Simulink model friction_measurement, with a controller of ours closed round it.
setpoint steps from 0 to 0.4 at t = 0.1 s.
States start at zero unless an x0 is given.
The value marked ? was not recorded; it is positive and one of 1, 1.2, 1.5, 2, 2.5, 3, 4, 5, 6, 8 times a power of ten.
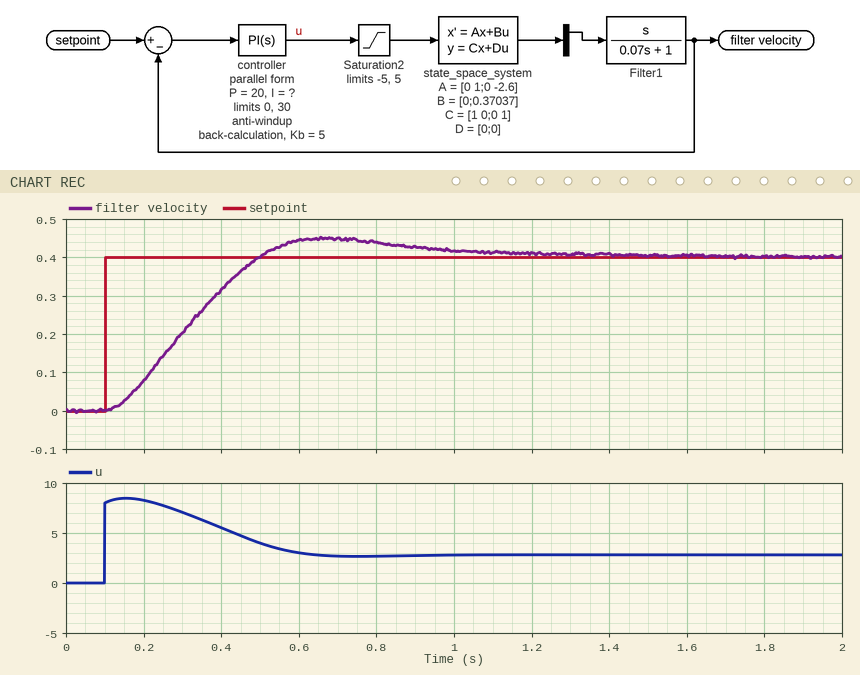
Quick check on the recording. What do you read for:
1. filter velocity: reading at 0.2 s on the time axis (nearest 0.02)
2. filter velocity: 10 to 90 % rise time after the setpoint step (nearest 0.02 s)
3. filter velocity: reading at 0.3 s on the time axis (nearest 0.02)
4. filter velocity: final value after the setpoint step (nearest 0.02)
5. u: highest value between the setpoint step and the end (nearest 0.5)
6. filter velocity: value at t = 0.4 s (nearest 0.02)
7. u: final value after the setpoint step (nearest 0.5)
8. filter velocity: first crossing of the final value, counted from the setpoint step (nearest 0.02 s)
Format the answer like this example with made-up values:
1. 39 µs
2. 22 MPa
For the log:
1. 0.08
2. 0.28 s
3. 0.20
4. 0.40
5. 8.5
6. 0.32
7. 3.0
8. 0.40 s
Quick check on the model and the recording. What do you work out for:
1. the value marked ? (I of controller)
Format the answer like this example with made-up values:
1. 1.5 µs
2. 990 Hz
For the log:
1. 50
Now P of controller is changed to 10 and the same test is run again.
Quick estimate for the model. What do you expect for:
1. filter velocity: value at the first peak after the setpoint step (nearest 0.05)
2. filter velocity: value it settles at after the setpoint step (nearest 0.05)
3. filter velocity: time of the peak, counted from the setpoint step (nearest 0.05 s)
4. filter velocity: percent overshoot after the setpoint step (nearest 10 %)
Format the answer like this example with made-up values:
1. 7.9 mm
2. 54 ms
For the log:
1. 0.45
2. 0.40
3. 0.65 s
4. 20 %
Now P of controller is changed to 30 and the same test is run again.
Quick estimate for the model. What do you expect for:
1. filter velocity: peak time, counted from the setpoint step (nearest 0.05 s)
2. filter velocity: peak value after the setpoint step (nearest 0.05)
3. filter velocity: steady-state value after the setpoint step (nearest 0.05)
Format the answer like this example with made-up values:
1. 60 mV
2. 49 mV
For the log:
1. 0.55 s
2. 0.45
3. 0.40
